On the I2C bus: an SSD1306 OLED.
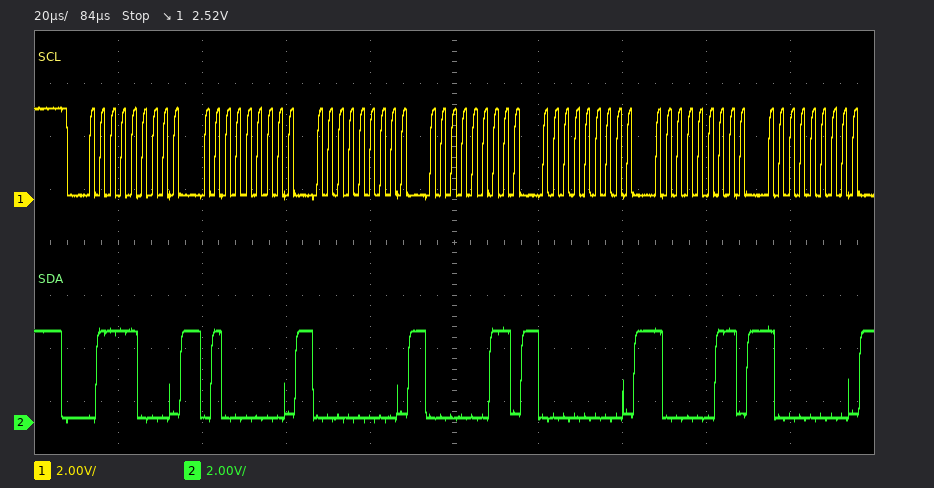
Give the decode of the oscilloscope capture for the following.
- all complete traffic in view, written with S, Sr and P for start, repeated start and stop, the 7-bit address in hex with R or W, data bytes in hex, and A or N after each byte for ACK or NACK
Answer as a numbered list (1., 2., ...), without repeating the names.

1. S 3CW A 40 A 00 A 03 A 00 A 83 A 80 A
